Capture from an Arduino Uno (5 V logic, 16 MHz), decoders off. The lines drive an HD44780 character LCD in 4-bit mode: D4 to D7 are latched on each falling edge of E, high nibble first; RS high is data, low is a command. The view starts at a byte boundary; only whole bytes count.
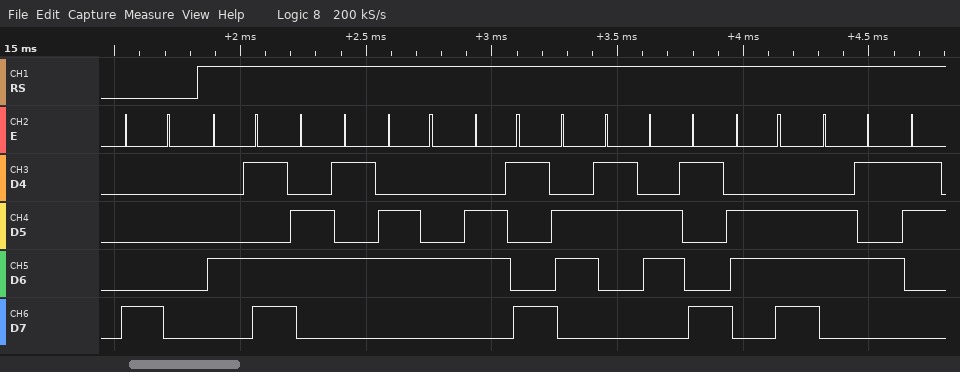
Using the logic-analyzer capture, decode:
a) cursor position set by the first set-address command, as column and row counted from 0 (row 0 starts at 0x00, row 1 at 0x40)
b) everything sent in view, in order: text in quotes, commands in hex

column 0, row 0
0x80 "Medicine"
